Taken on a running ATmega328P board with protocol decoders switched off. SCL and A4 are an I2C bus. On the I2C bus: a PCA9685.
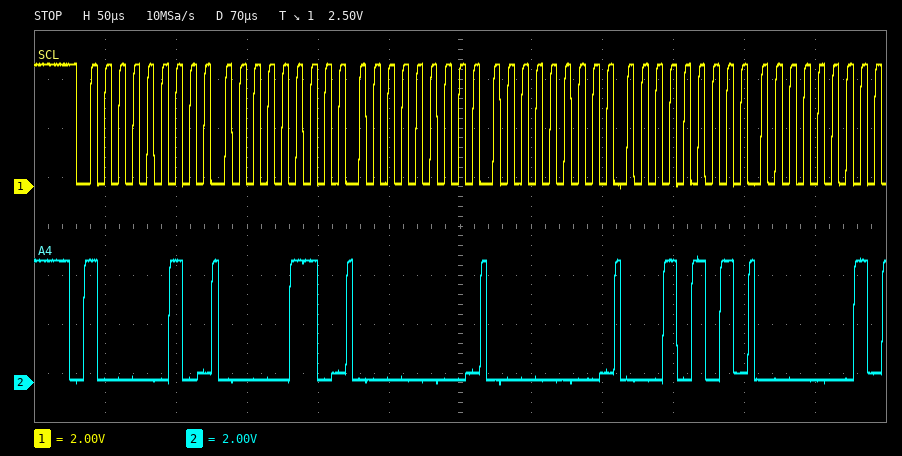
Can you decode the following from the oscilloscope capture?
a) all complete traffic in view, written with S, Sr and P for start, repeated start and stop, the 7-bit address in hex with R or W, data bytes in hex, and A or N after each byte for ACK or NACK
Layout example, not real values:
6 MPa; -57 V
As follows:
S 41W A 06 A 00 A 00 A 15 A 01 A
